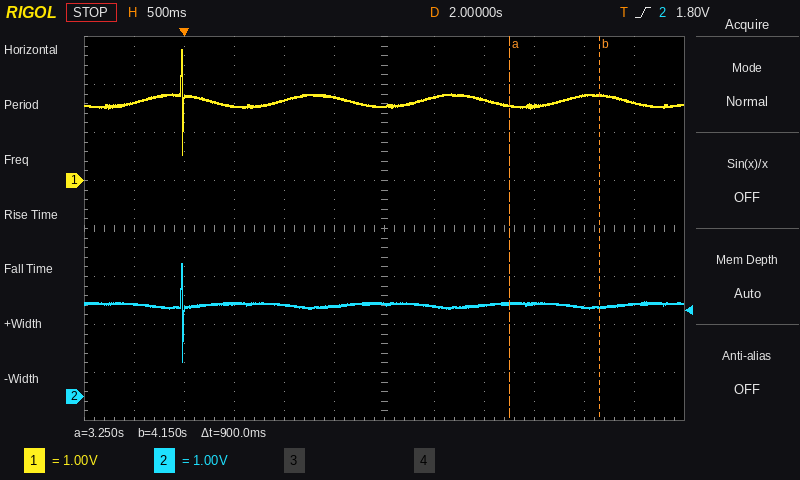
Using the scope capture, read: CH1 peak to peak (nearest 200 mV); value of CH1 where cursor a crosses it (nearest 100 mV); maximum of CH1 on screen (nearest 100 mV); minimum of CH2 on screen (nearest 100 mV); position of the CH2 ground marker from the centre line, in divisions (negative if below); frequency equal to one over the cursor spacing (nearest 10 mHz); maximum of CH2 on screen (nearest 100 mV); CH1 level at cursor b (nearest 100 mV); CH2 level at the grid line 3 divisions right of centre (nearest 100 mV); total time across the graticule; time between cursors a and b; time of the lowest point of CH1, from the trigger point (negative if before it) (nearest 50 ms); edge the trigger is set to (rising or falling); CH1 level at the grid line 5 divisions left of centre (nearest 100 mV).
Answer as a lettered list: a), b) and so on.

a) 2.2 V
b) 1.6 V
c) 2.7 V
d) 700 mV
e) -3.5 div
f) 1.11 Hz
g) 2.8 V
h) 1.8 V
i) 1.9 V
j) 6 s
k) 900 ms
l) 0 ms
m) rising
n) 1.6 V
